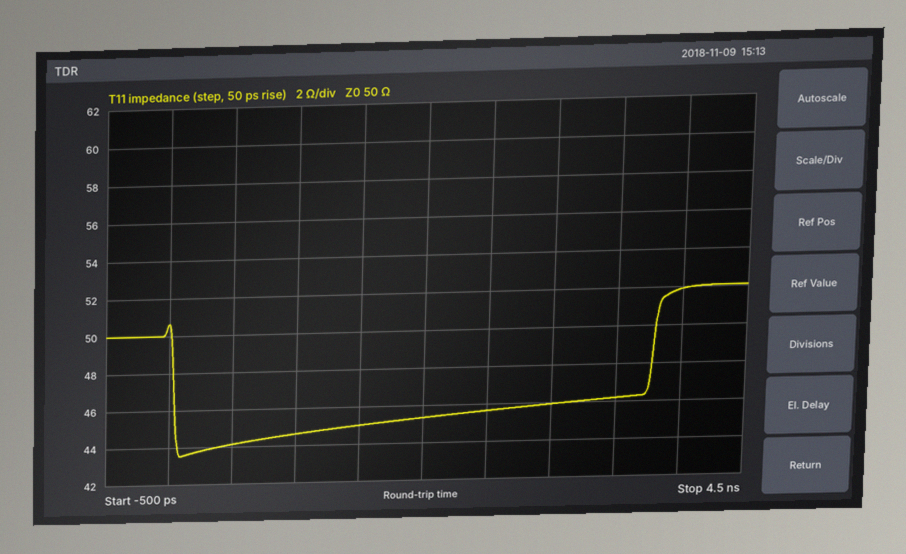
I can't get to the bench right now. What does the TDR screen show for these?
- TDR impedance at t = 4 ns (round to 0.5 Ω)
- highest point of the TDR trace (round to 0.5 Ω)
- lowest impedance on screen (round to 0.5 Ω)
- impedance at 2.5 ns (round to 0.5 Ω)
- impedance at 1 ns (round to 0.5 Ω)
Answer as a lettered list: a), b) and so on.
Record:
a) 52.0 Ω
b) 52.0 Ω
c) 43.5 Ω
d) 45.5 Ω
e) 44.5 Ω
